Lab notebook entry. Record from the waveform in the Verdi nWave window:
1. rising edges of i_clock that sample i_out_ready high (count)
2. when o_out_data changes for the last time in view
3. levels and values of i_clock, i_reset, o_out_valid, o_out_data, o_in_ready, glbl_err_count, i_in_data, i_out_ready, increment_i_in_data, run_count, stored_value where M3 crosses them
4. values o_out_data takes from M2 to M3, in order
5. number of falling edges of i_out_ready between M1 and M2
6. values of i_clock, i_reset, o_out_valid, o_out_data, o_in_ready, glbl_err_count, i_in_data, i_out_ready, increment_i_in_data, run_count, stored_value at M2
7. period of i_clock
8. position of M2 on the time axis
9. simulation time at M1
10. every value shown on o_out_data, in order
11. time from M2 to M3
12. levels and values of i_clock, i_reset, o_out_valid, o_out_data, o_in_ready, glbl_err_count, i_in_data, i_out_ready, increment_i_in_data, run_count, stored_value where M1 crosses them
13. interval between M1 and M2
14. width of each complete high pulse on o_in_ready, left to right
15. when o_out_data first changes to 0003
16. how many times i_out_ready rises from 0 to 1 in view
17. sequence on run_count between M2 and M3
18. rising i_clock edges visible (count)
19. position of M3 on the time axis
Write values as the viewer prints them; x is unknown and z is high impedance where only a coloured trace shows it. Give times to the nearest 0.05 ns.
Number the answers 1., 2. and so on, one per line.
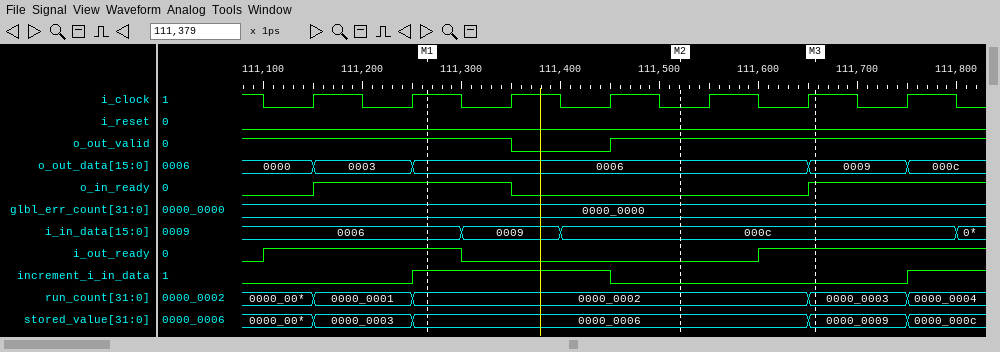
1. 4
2. 111.75 ns
3. i_clock=1, i_reset=0, o_out_valid=1, o_out_data=0009, o_in_ready=1, glbl_err_count=0000_0000, i_in_data=000c, i_out_ready=1, increment_i_in_data=0, run_count=0000_0003, stored_value=0000_0009
4. 0006, 0009
5. 1
6. i_clock=0, i_reset=0, o_out_valid=1, o_out_data=0006, o_in_ready=0, glbl_err_count=0000_0000, i_in_data=000c, i_out_ready=0, increment_i_in_data=0, run_count=0000_0002, stored_value=0000_0006
7. 0.1 ns
8. 111.5 ns
9. 111.25 ns
10. 0000, 0003, 0006, 0009, 000c
11. 0.15 ns
12. i_clock=1, i_reset=0, o_out_valid=1, o_out_data=0006, o_in_ready=1, glbl_err_count=0000_0000, i_in_data=0006, i_out_ready=1, increment_i_in_data=1, run_count=0000_0002, stored_value=0000_0006
13. 0.25 ns
14. 0.2 ns
15. 111.15 ns
16. 2
17. 0000_0002, 0000_0003
18. 7
19. 111.65 ns
